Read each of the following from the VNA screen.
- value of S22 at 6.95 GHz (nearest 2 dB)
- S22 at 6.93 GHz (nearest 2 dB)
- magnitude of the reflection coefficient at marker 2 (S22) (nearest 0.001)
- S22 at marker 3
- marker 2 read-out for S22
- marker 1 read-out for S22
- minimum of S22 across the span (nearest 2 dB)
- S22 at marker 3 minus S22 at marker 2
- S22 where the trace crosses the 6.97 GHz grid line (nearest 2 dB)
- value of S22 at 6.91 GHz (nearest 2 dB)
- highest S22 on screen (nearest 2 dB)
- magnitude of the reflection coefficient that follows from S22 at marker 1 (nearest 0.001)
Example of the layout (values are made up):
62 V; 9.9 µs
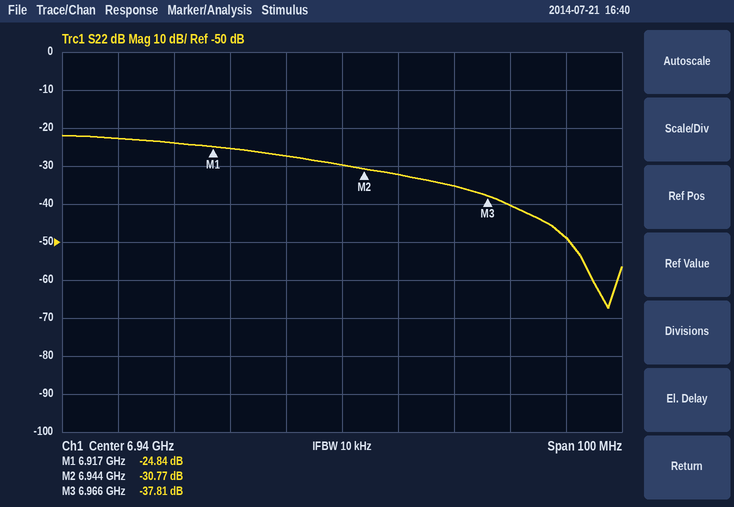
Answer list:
-32 dB; -28 dB; 0.029; -37.81 dB; -30.77 dB; -24.84 dB; -68 dB; -7.04 dB; -40 dB; -24 dB; -22 dB; 0.057
